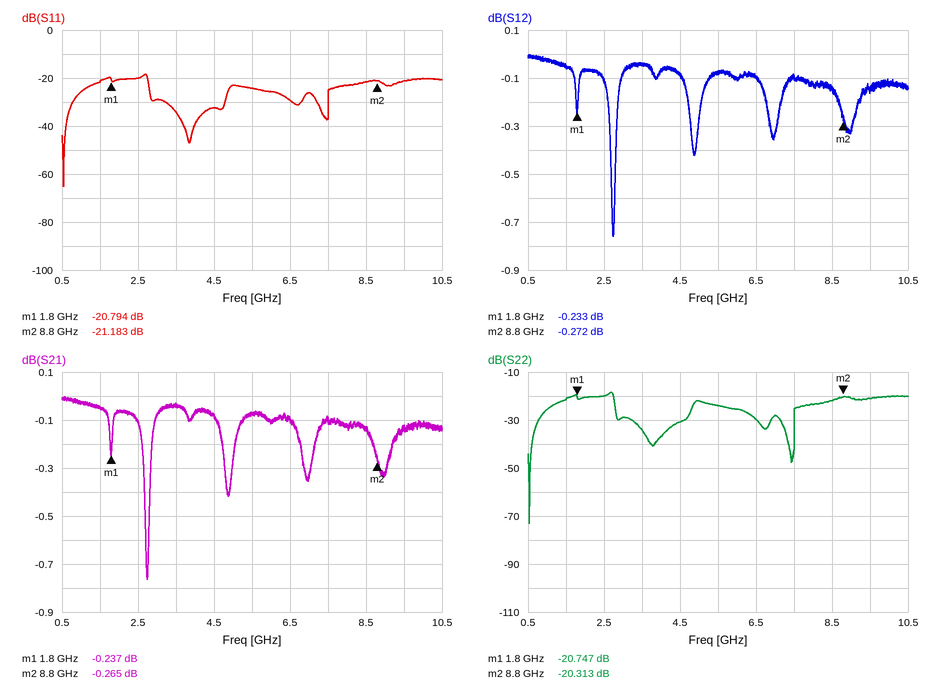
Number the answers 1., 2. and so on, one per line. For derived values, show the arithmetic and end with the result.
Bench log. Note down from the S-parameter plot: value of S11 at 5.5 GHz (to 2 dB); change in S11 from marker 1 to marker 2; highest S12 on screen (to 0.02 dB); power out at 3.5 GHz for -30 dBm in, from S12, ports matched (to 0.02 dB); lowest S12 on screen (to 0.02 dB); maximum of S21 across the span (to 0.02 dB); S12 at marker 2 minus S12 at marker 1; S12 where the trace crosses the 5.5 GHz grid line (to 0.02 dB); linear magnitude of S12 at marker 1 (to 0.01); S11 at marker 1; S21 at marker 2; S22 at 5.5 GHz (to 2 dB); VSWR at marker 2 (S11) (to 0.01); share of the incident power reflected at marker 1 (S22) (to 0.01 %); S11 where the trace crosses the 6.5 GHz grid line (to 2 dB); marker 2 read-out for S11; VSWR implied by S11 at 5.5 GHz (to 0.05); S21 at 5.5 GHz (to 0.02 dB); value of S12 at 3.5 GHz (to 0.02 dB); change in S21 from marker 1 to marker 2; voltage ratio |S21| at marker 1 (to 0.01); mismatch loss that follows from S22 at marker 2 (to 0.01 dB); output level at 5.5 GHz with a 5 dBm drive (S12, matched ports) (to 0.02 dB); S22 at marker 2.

1. -24 dB
2. -21.183 − (-20.794) = -0.389 dB
3. 0.00 dB
4. -30 dBm + (-0.04 dB) = -30.04 dBm
5. -0.76 dB
6. 0.00 dB
7. -0.272 − (-0.233) = -0.039 dB
8. -0.08 dB
9. 10^(-0.233/20) ≈ 0.97
10. -20.794 dB
11. -0.265 dB
12. -24 dB
13. (1 + 0.0873)/(1 − 0.0873) ≈ 1.19
14. 10^(-20.747/10) ≈ 0.84 %
15. -30 dB
16. -21.183 dB
17. |Γ| = 10^(-24/20) = 0.0631; VSWR = (1 + 0.0631)/(1 − 0.0631) ≈ 1.13, so 1.15 to the nearest 0.05
18. -0.08 dB
19. -0.04 dB
20. -0.265 − (-0.237) = -0.028 dB
21. 10^(-0.237/20) ≈ 0.97
22. −10 log10(1 − 10^(-20.313/10)) ≈ 0.04 dB
23. 5 dBm + (-0.08 dB) = 4.92 dBm
24. -20.313 dB
